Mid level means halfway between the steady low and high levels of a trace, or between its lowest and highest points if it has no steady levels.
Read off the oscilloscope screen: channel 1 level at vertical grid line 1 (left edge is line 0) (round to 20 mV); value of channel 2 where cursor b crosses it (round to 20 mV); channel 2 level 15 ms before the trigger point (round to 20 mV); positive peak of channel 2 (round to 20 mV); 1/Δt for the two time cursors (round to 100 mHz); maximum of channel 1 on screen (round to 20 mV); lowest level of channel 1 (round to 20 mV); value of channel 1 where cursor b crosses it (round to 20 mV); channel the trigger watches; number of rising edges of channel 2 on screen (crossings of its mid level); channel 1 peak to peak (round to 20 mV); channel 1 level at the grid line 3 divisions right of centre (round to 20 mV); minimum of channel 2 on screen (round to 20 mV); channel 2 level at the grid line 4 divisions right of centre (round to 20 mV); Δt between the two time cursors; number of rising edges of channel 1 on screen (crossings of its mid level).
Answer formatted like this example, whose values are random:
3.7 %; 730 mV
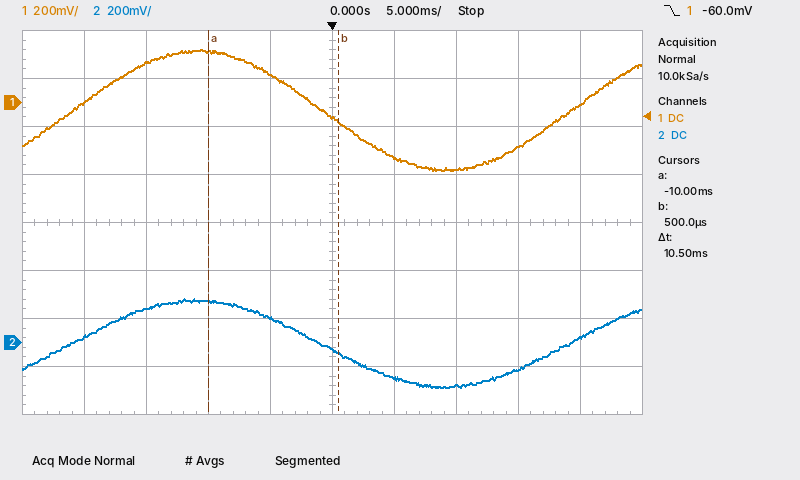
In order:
0 mV; -40 mV; 140 mV; 180 mV; 95.2 Hz; 220 mV; -280 mV; -80 mV; channel 1; 2; 500 mV; -180 mV; -180 mV; 20 mV; 10.5 ms; 2
